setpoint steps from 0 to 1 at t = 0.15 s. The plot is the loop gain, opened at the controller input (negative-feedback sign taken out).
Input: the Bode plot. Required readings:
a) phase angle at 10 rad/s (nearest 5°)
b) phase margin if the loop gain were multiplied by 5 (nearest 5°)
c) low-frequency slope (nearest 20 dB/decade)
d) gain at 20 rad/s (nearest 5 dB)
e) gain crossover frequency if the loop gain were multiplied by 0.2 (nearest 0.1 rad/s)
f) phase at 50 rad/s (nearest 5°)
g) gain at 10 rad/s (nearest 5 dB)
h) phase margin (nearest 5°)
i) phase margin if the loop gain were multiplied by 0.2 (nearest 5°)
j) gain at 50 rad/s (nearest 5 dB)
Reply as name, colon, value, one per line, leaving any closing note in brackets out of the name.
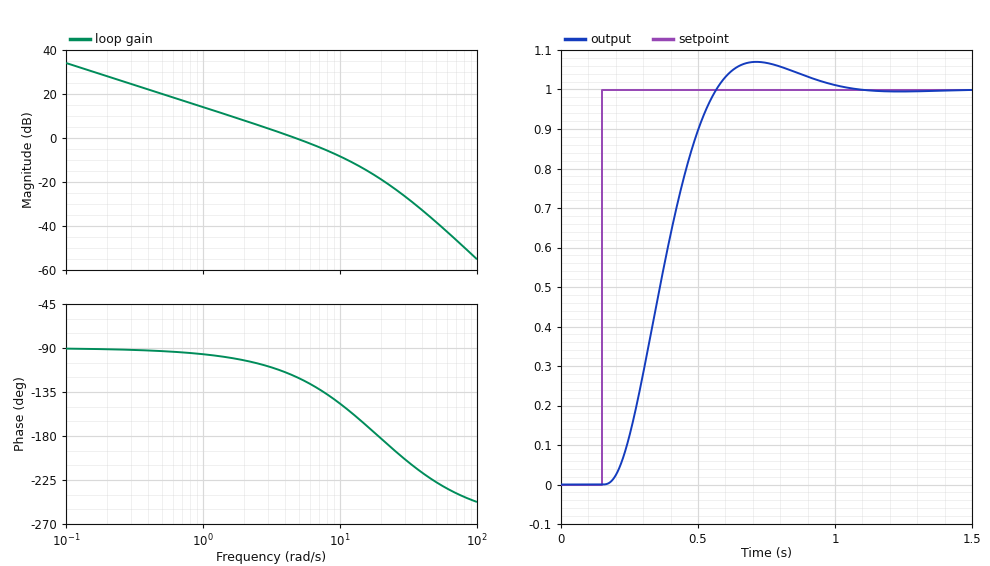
phase angle at 10 rad/s: -145°
phase margin if the loop gain were multiplied by 5: 15°
low-frequency slope: -20 dB/decade
gain at 20 rad/s: -20 dB
gain crossover frequency if the loop gain were multiplied by 0.2: 1.0 rad/s
phase at 50 rad/s: -225°
gain at 10 rad/s: -10 dB
phase margin: 60°
phase margin if the loop gain were multiplied by 0.2: 85°
gain at 50 rad/s: -40 dB
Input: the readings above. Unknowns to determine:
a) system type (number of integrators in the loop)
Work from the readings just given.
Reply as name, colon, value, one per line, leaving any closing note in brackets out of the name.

system type: 1
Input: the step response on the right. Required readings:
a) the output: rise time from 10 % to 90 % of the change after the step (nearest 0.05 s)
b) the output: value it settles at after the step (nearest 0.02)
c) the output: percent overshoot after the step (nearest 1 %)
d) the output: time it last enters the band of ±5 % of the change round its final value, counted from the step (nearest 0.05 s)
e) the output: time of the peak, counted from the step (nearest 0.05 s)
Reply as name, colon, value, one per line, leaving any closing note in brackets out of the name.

the output: rise time from 10 % to 90 % of the change after the step: 0.25 s
the output: value it settles at after the step: 1.00
the output: percent overshoot after the step: 7 %
the output: time it last enters the band of ±5 % of the change round its final value, counted from the step: 0.70 s
the output: time of the peak, counted from the step: 0.55 s
